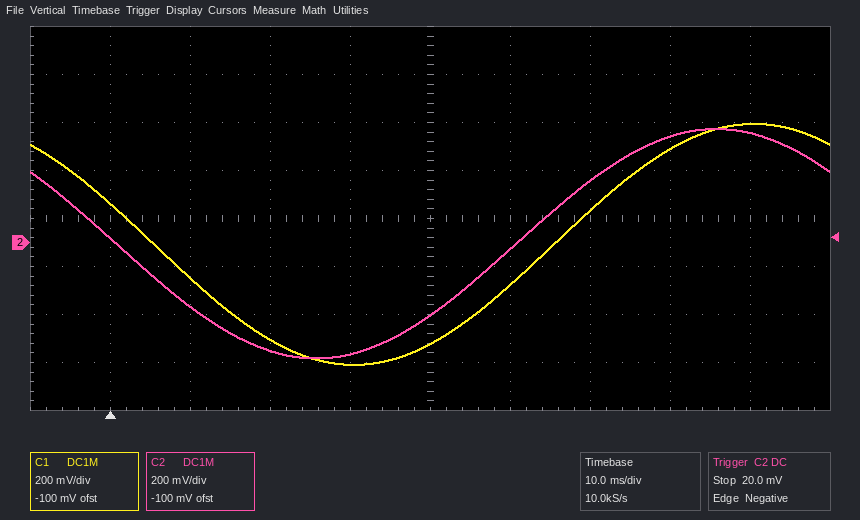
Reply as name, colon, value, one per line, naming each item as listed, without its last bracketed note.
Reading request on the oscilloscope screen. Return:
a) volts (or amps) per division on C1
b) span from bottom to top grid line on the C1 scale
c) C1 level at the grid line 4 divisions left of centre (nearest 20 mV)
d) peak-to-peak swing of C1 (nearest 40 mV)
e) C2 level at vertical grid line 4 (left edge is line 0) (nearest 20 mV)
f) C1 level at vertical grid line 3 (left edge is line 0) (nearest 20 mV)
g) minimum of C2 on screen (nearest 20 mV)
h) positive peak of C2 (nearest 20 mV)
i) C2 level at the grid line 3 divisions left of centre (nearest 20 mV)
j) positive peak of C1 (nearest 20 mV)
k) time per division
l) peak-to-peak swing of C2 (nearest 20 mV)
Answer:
volts (or amps) per division on C1: 200 mV
span from bottom to top grid line on the C1 scale: 1.6 V
C1 level at the grid line 4 divisions left of centre: 160 mV
peak-to-peak swing of C1: 1.00 V
C2 level at vertical grid line 4 (left edge is line 0): -460 mV
C1 level at vertical grid line 3 (left edge is line 0): -400 mV
minimum of C2 on screen: -480 mV
positive peak of C2: 480 mV
C2 level at the grid line 3 divisions left of centre: -260 mV
positive peak of C1: 500 mV
time per division: 10 ms
peak-to-peak swing of C2: 960 mV
